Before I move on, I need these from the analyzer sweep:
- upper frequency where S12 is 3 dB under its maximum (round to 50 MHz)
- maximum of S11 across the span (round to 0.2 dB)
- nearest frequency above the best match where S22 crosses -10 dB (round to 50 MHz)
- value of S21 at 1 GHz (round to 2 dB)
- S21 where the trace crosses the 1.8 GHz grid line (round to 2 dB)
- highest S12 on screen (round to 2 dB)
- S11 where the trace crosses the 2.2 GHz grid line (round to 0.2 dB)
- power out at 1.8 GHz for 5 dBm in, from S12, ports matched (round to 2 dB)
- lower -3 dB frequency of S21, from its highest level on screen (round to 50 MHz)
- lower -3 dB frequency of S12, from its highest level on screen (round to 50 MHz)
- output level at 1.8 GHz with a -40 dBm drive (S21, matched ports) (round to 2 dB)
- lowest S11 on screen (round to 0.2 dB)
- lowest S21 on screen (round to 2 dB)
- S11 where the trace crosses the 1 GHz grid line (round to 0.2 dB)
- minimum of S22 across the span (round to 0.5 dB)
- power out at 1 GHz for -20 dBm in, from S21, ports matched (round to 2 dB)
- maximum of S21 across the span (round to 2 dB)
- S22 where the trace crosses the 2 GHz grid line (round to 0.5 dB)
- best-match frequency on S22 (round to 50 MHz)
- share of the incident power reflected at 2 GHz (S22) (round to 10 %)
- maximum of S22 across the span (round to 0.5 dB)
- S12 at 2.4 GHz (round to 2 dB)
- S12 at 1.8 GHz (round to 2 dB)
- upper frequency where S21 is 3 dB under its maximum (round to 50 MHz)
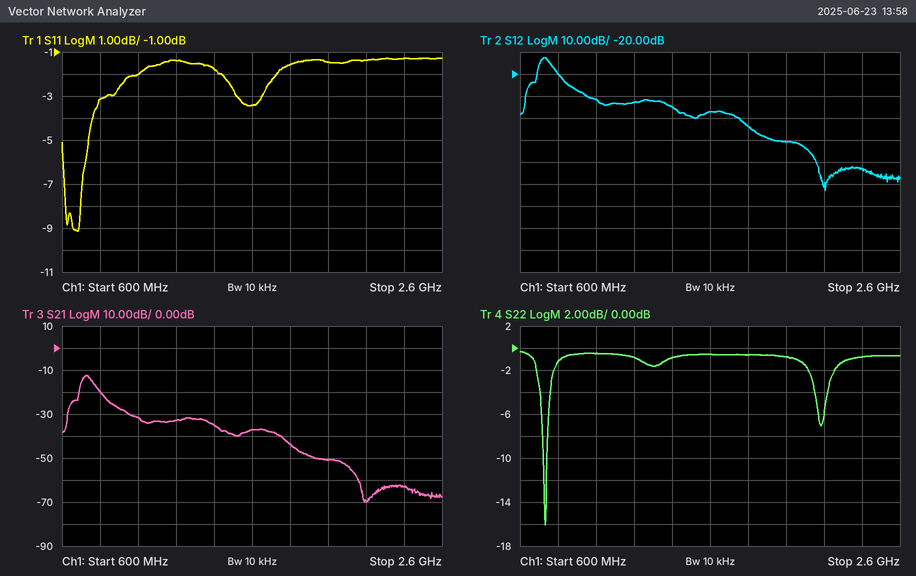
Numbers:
750 MHz
-1.2 dB
750 MHz
-32 dB
-44 dB
-12 dB
-1.4 dB
-38 dBm
700 MHz
700 MHz
-84 dBm
-9.2 dB
-70 dB
-2.0 dB
-16.0 dB
-52 dBm
-12 dB
-1.0 dB
750 MHz
80 %
-0.5 dB
-64 dB
-44 dB
750 MHz
